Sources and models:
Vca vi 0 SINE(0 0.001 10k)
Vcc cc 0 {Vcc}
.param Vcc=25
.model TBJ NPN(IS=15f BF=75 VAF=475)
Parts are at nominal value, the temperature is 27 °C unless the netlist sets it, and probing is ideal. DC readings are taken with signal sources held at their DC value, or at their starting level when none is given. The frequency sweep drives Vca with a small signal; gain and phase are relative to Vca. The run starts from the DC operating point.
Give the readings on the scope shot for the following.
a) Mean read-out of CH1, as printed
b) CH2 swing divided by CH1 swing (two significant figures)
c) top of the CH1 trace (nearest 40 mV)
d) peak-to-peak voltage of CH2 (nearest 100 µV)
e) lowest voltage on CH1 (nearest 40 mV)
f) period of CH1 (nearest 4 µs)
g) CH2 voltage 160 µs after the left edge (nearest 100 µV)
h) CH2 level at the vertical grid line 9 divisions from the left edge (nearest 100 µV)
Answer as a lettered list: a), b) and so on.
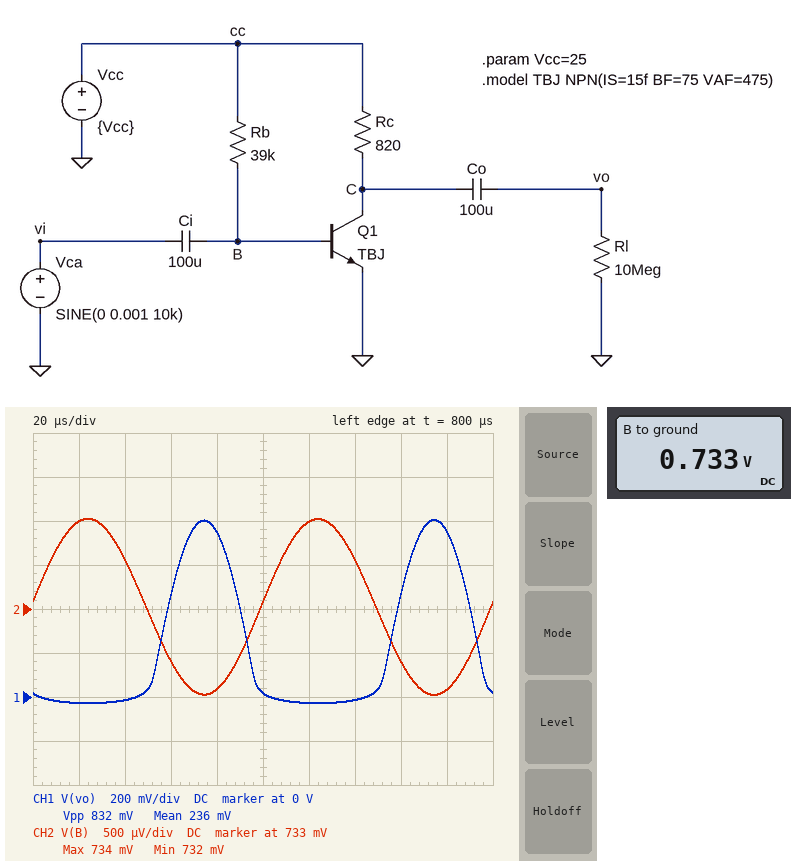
a) 236 mV
b) 0.0024
c) 800 mV
d) 2.0 mV
e) -40 mV
f) 100 µs
g) 732.4 mV
h) 732.1 mV
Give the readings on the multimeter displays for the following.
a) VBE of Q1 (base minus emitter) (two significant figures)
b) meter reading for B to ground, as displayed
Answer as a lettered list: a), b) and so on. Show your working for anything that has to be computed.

a) 733 mV = 730 mV
b) 0.733 V
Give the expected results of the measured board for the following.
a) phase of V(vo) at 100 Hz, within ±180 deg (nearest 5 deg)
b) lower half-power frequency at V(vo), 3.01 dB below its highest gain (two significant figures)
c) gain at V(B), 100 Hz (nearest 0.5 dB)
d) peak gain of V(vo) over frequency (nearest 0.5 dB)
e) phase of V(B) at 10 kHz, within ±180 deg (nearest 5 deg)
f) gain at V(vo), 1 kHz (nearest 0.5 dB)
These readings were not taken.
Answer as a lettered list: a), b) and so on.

a) -95 deg
b) 900 Hz
c) -19.0 dB
d) 36.5 dB
e) 5 deg
f) 34.0 dB
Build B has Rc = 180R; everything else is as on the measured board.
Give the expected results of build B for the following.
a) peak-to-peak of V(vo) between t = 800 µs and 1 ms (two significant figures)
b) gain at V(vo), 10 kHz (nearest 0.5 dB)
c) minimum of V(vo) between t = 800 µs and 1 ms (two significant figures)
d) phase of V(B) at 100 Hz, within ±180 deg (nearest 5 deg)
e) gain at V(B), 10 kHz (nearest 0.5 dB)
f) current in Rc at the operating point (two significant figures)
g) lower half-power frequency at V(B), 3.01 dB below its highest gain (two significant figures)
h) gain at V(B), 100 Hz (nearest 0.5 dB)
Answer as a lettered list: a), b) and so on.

a) 660 mV
b) 50.5 dB
c) -330 mV
d) 20 deg
e) 0 dB
f) 48 mA
g) 38 Hz
h) -0.5 dB
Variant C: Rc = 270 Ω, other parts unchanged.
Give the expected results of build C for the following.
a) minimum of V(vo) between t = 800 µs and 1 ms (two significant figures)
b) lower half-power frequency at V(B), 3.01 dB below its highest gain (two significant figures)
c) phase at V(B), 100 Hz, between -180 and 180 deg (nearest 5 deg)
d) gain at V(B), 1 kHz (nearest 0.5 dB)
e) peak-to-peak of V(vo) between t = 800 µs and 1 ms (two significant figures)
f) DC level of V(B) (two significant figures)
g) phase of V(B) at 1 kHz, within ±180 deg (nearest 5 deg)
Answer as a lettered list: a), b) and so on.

a) -490 mV
b) 38 Hz
c) 20 deg
d) 0 dB
e) 970 mV
f) 740 mV
g) 0 deg
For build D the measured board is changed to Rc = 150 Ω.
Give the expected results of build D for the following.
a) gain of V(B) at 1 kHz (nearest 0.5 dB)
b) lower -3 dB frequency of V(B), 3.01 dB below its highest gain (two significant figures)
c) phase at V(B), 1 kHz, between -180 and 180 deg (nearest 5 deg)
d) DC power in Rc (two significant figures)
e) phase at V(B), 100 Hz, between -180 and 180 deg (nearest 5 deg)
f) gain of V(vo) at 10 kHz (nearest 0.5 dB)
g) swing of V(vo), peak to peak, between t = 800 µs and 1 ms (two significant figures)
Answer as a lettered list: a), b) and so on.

a) 0 dB
b) 38 Hz
c) 0 deg
d) 350 mW
e) 20 deg
f) 49.0 dB
g) 550 mV
